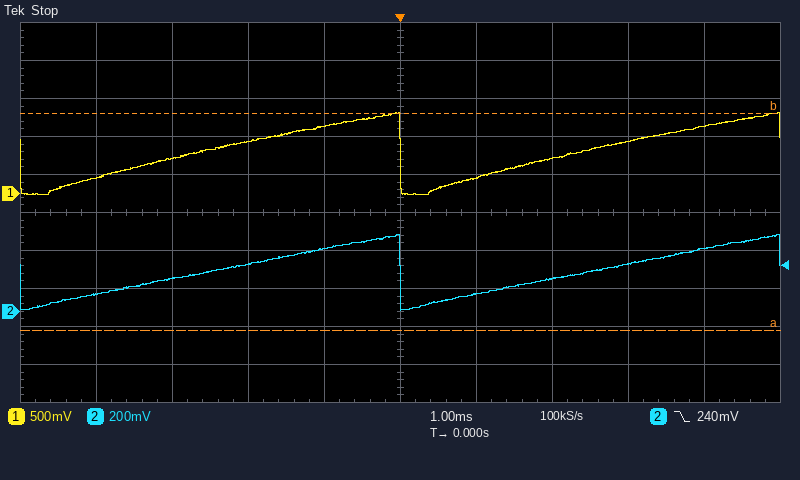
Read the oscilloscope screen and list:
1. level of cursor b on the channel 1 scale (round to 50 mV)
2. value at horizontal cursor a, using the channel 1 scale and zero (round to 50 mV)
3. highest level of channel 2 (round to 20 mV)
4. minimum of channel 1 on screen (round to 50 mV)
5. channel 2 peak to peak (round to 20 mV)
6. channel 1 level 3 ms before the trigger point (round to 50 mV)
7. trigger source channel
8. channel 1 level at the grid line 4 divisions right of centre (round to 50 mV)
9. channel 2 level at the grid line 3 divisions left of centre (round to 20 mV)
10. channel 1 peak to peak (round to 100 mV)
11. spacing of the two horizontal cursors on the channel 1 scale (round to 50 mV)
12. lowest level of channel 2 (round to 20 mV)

1.05 V
-1.80 V
400 mV
0 mV
400 mV
450 mV
channel 2
900 mV
180 mV
1.10 V
2.85 V
0 mV
